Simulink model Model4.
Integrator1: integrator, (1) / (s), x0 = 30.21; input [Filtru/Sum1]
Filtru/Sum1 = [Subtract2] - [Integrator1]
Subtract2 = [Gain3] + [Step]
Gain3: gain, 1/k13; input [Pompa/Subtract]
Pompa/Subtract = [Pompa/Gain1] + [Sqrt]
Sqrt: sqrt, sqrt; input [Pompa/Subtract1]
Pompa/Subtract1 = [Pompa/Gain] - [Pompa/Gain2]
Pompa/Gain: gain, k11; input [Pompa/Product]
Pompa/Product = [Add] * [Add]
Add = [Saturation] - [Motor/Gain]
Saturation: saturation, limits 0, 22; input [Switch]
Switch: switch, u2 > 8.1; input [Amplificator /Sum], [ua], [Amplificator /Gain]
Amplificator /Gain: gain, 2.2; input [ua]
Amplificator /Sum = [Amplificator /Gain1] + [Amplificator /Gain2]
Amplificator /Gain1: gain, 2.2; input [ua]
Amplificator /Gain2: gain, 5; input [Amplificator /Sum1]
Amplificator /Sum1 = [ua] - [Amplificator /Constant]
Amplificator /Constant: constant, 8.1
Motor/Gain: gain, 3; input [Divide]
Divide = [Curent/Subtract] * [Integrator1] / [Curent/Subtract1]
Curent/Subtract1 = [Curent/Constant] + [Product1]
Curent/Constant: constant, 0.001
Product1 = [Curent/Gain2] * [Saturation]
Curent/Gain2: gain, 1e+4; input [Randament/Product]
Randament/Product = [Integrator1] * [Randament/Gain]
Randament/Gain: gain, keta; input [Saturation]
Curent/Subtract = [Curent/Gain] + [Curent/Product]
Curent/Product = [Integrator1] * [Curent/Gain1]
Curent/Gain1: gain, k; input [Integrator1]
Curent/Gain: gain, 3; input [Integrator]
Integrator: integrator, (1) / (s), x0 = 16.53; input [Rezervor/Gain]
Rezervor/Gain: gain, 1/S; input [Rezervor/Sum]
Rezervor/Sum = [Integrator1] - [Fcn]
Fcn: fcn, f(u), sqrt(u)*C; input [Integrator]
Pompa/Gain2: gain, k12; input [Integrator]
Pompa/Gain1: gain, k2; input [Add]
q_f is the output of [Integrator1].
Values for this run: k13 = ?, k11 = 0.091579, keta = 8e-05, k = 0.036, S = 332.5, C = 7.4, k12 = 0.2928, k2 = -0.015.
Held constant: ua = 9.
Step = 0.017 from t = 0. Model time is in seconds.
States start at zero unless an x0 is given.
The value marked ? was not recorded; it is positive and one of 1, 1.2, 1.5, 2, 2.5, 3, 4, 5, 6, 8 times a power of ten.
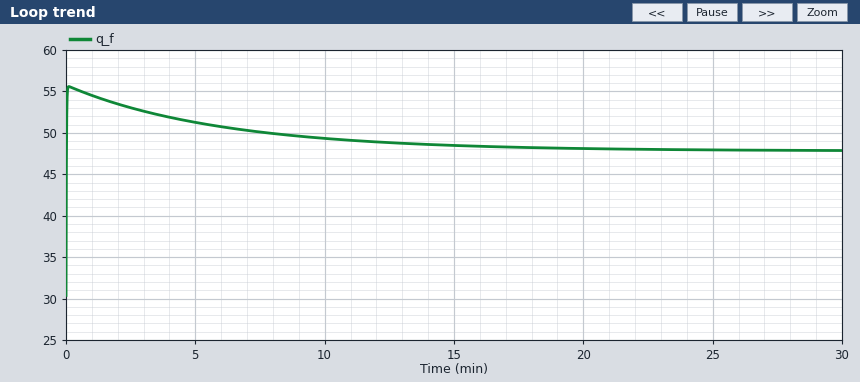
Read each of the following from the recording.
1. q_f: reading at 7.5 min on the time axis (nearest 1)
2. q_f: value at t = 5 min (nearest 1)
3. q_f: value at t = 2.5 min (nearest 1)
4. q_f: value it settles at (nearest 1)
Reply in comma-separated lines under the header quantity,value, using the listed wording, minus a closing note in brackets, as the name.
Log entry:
quantity,value
q_f: reading at 7.5 min on the time axis,50
q_f: value at t = 5 min,51
q_f: value at t = 2.5 min,53
q_f: value it settles at,48
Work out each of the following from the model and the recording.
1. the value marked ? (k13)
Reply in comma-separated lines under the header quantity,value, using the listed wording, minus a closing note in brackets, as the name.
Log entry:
quantity,value
the value marked ?,0.1
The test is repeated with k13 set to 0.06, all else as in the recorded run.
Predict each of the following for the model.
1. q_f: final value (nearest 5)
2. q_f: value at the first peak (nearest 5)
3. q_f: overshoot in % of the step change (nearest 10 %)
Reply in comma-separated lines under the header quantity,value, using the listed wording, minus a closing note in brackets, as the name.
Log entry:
quantity,value
q_f: final value,60
q_f: value at the first peak,85
q_f: overshoot in % of the step change,90 %
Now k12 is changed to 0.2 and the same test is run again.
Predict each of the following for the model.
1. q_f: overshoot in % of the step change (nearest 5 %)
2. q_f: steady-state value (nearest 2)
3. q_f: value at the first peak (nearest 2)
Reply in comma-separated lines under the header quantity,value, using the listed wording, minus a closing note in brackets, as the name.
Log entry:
quantity,value
q_f: overshoot in % of the step change,35 %
q_f: steady-state value,50
q_f: value at the first peak,56
